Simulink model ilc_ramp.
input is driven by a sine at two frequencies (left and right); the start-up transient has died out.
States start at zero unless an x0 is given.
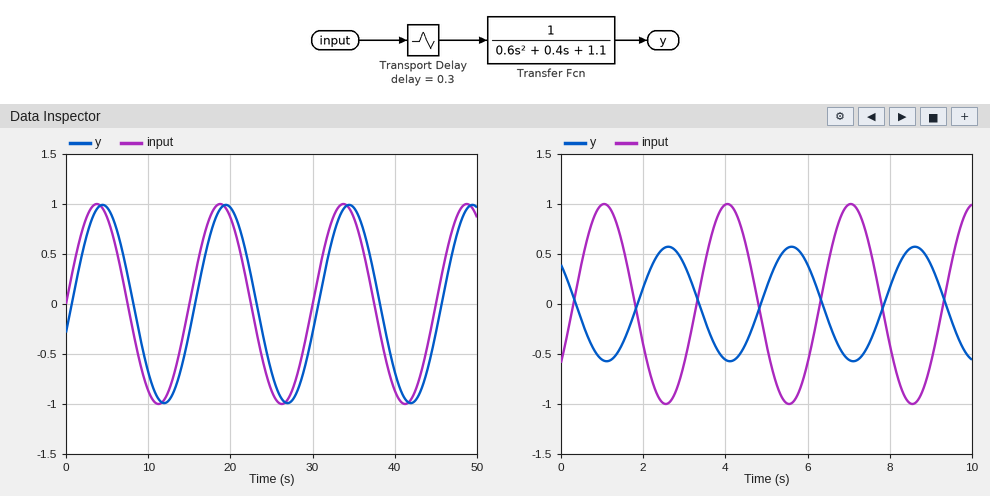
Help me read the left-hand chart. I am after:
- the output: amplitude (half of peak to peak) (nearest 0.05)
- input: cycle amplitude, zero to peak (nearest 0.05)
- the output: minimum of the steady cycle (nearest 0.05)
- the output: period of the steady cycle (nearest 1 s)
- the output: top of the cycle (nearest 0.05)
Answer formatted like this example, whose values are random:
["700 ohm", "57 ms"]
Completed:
["1.00", "1.00", "-1.00", "15 s", "1.00"]
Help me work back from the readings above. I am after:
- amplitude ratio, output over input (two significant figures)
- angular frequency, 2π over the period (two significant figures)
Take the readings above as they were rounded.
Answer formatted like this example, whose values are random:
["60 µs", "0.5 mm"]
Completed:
["1.0", "0.42 rad/s"]
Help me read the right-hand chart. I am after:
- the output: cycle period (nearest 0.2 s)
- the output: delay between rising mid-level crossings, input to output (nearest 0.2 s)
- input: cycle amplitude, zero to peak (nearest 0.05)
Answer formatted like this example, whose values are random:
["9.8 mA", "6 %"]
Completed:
["3.0 s", "1.6 s", "1.00"]
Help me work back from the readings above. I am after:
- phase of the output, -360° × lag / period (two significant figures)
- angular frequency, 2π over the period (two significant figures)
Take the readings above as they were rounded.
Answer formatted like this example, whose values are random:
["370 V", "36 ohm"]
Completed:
["-190°", "2.1 rad/s"]
